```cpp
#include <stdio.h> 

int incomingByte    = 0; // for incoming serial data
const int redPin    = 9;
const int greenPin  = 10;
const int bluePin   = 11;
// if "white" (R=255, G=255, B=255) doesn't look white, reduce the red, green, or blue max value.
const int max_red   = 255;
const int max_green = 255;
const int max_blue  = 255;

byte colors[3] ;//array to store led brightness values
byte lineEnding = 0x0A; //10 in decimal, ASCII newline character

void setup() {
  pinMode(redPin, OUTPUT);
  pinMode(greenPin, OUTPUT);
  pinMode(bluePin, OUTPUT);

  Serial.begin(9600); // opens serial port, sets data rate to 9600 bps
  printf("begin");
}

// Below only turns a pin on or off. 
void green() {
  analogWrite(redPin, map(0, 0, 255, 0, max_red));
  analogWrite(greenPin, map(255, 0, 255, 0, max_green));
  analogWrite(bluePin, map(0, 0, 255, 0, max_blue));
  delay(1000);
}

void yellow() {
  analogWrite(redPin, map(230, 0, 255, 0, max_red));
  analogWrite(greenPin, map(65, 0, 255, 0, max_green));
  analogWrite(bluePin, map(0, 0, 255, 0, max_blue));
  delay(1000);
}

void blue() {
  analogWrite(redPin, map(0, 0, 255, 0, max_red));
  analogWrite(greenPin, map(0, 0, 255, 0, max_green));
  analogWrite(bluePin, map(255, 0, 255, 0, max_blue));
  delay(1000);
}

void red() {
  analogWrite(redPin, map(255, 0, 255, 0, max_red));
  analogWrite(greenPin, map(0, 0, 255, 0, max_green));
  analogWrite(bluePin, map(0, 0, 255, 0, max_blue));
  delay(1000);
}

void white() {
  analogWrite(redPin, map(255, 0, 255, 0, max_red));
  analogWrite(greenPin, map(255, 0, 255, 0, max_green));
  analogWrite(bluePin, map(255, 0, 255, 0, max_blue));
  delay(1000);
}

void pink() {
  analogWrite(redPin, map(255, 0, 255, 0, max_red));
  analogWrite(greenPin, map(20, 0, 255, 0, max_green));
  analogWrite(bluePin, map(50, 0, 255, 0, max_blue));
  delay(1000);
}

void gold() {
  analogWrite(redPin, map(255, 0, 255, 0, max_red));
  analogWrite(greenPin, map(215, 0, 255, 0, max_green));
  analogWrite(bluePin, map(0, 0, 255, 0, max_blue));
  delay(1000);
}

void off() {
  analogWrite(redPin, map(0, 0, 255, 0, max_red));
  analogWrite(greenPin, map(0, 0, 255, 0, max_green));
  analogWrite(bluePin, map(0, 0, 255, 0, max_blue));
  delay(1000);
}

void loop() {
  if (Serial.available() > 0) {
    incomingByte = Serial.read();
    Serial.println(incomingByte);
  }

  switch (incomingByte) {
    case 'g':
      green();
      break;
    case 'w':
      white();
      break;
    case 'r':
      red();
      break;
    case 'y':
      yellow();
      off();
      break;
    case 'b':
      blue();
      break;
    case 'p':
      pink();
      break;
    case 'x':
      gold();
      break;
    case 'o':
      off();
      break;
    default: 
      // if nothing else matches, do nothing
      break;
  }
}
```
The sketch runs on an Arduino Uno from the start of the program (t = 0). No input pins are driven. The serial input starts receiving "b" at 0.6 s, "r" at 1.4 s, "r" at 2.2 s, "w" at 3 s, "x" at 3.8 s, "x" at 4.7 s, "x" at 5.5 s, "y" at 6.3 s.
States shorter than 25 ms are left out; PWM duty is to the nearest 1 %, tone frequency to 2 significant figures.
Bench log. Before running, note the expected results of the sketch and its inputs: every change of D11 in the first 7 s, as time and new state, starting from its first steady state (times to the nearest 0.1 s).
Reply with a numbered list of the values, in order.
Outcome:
1. 0 s low; 0.6 s high; 1.6 s low; 3.6 s high; 4.6 s low
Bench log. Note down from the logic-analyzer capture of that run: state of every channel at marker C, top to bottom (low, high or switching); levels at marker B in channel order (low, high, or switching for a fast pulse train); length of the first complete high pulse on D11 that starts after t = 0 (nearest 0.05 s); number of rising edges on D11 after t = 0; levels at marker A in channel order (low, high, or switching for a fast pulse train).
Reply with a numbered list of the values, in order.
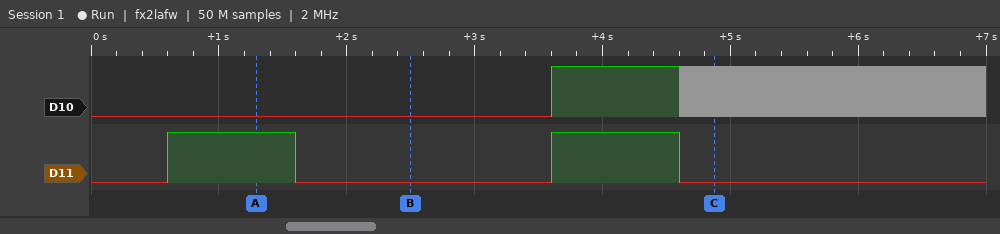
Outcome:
1. D10 switching, D11 low
2. D10 low, D11 low
3. 1.00 s
4. 2
5. D10 low, D11 high
